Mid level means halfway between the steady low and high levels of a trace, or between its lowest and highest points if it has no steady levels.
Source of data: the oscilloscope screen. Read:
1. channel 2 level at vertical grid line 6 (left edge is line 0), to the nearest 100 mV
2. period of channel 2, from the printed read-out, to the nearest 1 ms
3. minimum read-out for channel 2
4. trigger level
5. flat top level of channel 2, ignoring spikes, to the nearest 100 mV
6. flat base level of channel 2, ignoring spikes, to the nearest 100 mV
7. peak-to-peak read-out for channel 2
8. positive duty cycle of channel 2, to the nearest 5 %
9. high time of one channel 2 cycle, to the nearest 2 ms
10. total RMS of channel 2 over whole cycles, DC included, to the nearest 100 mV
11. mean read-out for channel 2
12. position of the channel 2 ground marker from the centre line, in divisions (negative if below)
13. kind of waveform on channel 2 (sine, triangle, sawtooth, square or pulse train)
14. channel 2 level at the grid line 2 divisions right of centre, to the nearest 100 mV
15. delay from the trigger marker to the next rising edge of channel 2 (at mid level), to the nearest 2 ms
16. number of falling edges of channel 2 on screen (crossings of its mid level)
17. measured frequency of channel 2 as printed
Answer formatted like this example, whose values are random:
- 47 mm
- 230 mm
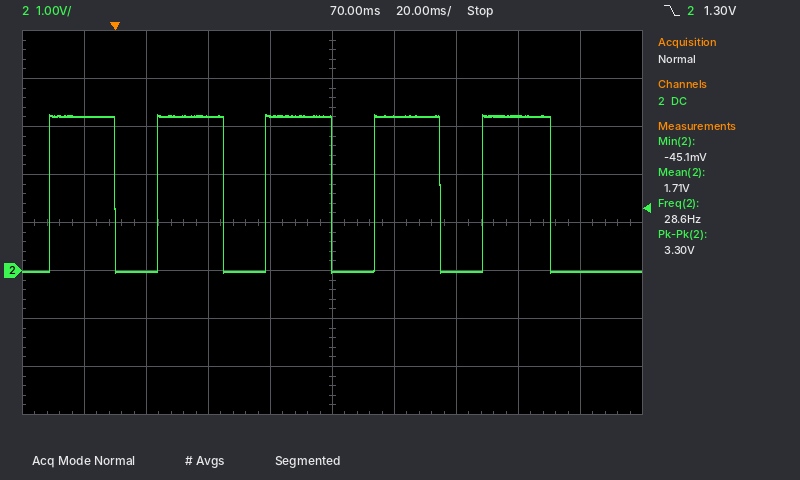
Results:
- 3.2 V
- 35 ms
- -45.1 mV
- 1.30 V
- 3.2 V
- 0.0 V
- 3.30 V
- 60 %
- 22 ms
- 2.5 V
- 1.71 V
- -1.0 div
- pulse train
- 0.0 V
- 14 ms
- 5
- 28.6 Hz
